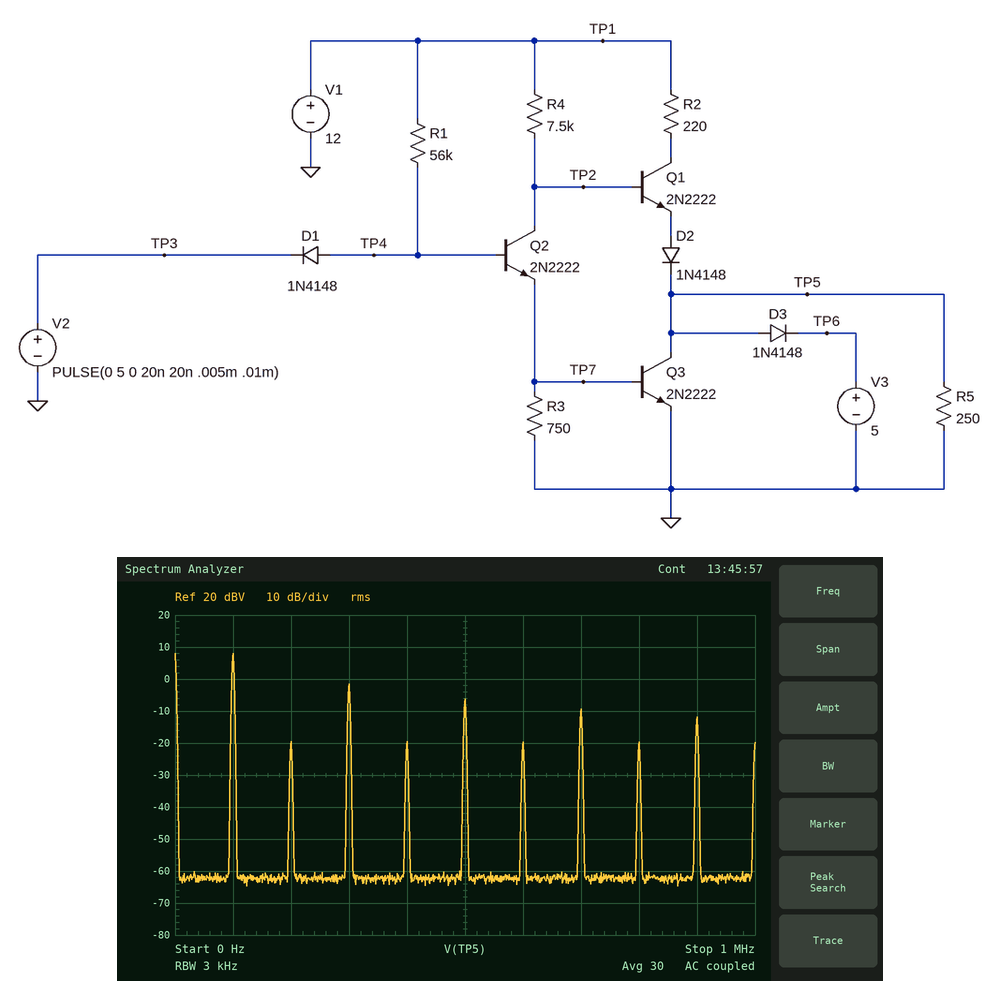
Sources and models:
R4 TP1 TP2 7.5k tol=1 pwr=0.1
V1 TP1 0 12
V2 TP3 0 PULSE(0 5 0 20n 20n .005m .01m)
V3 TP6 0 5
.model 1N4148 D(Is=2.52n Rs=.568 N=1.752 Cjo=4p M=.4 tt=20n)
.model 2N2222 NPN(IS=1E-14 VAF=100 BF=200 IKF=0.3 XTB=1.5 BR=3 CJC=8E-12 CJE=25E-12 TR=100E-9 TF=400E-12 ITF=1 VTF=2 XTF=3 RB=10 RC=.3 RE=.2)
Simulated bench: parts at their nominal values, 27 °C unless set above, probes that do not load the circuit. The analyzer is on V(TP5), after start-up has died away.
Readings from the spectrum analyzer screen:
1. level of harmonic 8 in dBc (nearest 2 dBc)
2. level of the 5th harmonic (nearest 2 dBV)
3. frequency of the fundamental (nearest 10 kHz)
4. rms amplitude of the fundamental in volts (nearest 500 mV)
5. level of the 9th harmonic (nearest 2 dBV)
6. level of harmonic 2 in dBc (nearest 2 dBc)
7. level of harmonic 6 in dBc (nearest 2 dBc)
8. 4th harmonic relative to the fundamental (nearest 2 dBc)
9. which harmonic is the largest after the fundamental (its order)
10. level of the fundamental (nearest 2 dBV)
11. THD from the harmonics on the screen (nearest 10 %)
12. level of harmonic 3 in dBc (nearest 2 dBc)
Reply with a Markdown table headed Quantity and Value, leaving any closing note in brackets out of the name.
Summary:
| Quantity | Value |
|---|---|
| level of harmonic 8 in dBc | -28 dBc |
| level of the 5th harmonic | -6 dBV |
| frequency of the fundamental | 100 kHz |
| rms amplitude of the fundamental in volts | 2.5 V |
| level of the 9th harmonic | -12 dBV |
| level of harmonic 2 in dBc | -28 dBc |
| level of harmonic 6 in dBc | -28 dBc |
| 4th harmonic relative to the fundamental | -28 dBc |
| which harmonic is the largest after the fundamental | 3 |
| level of the fundamental | 8 dBV |
| THD from the harmonics on the screen | 40 % |
| level of harmonic 3 in dBc | -10 dBc |
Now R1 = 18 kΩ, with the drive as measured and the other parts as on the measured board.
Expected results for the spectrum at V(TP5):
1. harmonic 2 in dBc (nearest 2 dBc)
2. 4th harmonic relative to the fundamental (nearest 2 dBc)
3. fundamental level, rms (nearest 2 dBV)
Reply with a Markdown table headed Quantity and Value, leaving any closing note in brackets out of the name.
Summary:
| Quantity | Value |
|---|---|
| harmonic 2 in dBc | -24 dBc |
| 4th harmonic relative to the fundamental | -24 dBc |
| fundamental level, rms | 8 dBV |
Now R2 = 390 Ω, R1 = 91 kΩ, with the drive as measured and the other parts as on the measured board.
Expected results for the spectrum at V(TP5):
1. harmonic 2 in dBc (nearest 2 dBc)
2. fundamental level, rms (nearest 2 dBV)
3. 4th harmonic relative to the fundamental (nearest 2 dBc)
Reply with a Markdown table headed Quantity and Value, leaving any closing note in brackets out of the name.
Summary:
| Quantity | Value |
|---|---|
| harmonic 2 in dBc | -30 dBc |
| fundamental level, rms | 6 dBV |
| 4th harmonic relative to the fundamental | -30 dBc |
